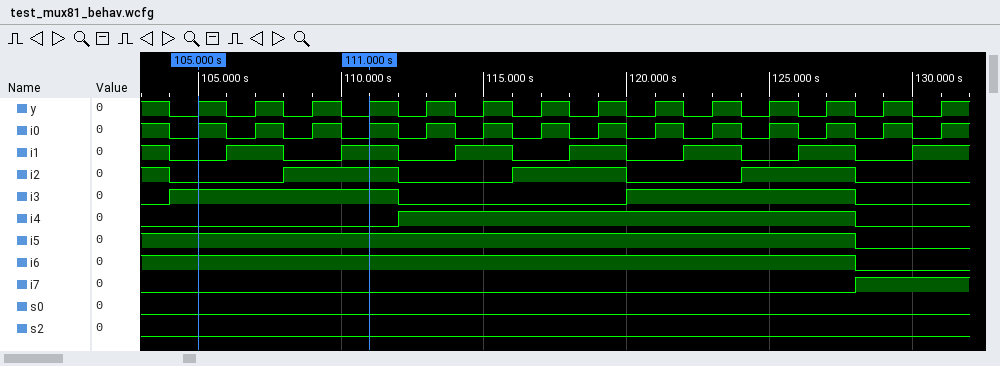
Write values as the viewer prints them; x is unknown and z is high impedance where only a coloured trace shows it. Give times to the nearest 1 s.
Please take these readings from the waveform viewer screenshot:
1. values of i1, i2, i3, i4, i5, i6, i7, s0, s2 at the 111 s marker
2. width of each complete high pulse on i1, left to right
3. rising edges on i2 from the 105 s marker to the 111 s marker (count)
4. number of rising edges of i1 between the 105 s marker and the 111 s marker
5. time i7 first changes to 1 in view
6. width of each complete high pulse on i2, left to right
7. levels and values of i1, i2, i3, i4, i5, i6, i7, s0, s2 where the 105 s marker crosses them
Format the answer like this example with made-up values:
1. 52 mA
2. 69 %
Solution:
1. i1=1, i2=1, i3=1, i4=0, i5=1, i6=1, i7=0, s0=0, s2=0
2. 2 s, 2 s, 2 s, 2 s, 2 s, 2 s
3. 1
4. 2
5. 128 s
6. 4 s, 4 s, 4 s
7. i1=0, i2=0, i3=1, i4=0, i5=1, i6=1, i7=0, s0=0, s2=0
